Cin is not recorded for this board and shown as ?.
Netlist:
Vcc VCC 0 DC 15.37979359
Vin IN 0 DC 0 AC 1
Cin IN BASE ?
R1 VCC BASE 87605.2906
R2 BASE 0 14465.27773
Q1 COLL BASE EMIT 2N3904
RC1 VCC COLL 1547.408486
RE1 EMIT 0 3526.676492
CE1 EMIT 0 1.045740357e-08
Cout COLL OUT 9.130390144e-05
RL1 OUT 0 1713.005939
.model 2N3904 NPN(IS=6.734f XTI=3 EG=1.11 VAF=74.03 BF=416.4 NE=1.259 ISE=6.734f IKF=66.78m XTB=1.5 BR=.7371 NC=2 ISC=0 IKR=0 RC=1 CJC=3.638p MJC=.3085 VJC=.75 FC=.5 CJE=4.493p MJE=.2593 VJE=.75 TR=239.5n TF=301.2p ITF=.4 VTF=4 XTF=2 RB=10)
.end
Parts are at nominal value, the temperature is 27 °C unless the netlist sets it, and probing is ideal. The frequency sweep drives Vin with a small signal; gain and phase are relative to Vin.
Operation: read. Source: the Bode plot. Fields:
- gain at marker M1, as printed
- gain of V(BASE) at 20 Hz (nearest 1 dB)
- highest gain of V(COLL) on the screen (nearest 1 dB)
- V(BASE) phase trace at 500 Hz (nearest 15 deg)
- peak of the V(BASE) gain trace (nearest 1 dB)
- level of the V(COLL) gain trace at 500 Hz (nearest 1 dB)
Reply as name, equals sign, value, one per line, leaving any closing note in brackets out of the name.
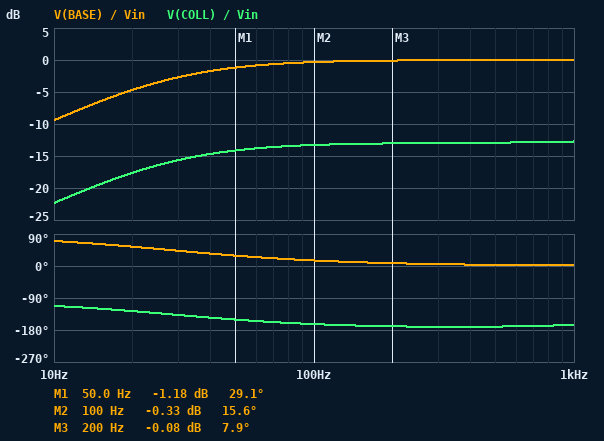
gain at marker M1, as printed = -1.18 dB
gain of V(BASE) at 20 Hz = -5 dB
highest gain of V(COLL) on the screen = -13 dB
V(BASE) phase trace at 500 Hz = 0 deg
peak of the V(BASE) gain trace = 0 dB
level of the V(COLL) gain trace at 500 Hz = -13 dB
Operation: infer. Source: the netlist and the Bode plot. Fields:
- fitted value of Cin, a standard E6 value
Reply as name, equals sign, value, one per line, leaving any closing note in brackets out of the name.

fitted value of Cin, a standard E6 value = 470 nF
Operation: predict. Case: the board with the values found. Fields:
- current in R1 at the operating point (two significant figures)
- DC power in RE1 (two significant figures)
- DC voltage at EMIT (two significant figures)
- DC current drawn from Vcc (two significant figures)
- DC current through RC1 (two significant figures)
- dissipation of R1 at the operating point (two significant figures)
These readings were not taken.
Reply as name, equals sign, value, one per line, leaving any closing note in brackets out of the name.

current in R1 at the operating point = 150 µA
DC power in RE1 = 640 µW
DC voltage at EMIT = 1.5 V
DC current drawn from Vcc = 570 µA
DC current through RC1 = 420 µA
dissipation of R1 at the operating point = 2.0 mW
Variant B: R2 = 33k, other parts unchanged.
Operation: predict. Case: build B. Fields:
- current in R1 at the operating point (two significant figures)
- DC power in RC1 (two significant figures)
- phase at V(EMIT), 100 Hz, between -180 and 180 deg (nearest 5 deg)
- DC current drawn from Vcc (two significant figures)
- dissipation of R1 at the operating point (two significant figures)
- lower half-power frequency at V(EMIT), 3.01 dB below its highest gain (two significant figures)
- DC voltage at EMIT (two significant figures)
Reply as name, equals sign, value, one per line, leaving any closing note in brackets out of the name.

current in R1 at the operating point = 130 µA
DC power in RC1 = 1.4 mW
phase at V(EMIT), 100 Hz, between -180 and 180 deg = 10 deg
DC current drawn from Vcc = 1.1 mA
dissipation of R1 at the operating point = 1.5 mW
lower half-power frequency at V(EMIT), 3.01 dB below its highest gain = 15 Hz
DC voltage at EMIT = 3.4 V
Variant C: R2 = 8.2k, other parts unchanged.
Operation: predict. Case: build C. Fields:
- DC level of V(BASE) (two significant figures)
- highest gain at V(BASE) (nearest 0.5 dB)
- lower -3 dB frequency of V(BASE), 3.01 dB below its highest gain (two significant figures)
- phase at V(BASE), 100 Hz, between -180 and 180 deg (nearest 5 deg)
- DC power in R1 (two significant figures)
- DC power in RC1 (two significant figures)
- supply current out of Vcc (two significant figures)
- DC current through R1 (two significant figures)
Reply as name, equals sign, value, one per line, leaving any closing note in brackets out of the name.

DC level of V(BASE) = 1.3 V
highest gain at V(BASE) = 0 dB
lower -3 dB frequency of V(BASE), 3.01 dB below its highest gain = 46 Hz
phase at V(BASE), 100 Hz, between -180 and 180 deg = 25 deg
DC power in R1 = 2.3 mW
DC power in RC1 = 58 µW
supply current out of Vcc = 350 µA
DC current through R1 = 160 µA
